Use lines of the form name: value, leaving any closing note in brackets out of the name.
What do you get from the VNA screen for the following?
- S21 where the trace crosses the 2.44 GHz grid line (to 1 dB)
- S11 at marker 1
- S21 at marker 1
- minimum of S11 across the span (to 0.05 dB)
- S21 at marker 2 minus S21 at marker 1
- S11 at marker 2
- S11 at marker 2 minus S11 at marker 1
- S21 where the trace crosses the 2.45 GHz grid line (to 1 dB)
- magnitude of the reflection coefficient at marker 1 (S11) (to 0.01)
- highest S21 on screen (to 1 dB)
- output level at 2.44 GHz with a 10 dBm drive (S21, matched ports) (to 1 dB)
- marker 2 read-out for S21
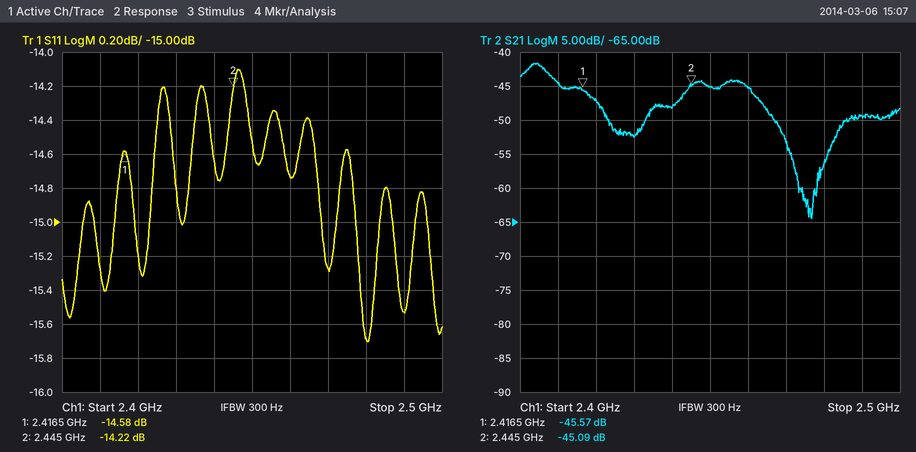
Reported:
S21 where the trace crosses the 2.44 GHz grid line: -48 dB
S11 at marker 1: -14.58 dB
S21 at marker 1: -45.57 dB
minimum of S11 across the span: -15.70 dB
S21 at marker 2 minus S21 at marker 1: 0.48 dB
S11 at marker 2: -14.22 dB
S11 at marker 2 minus S11 at marker 1: 0.36 dB
S21 where the trace crosses the 2.45 GHz grid line: -45 dB
magnitude of the reflection coefficient at marker 1 (S11): 0.19
highest S21 on screen: -42 dB
output level at 2.44 GHz with a 10 dBm drive (S21, matched ports): -38 dBm
marker 2 read-out for S21: -45.09 dB
